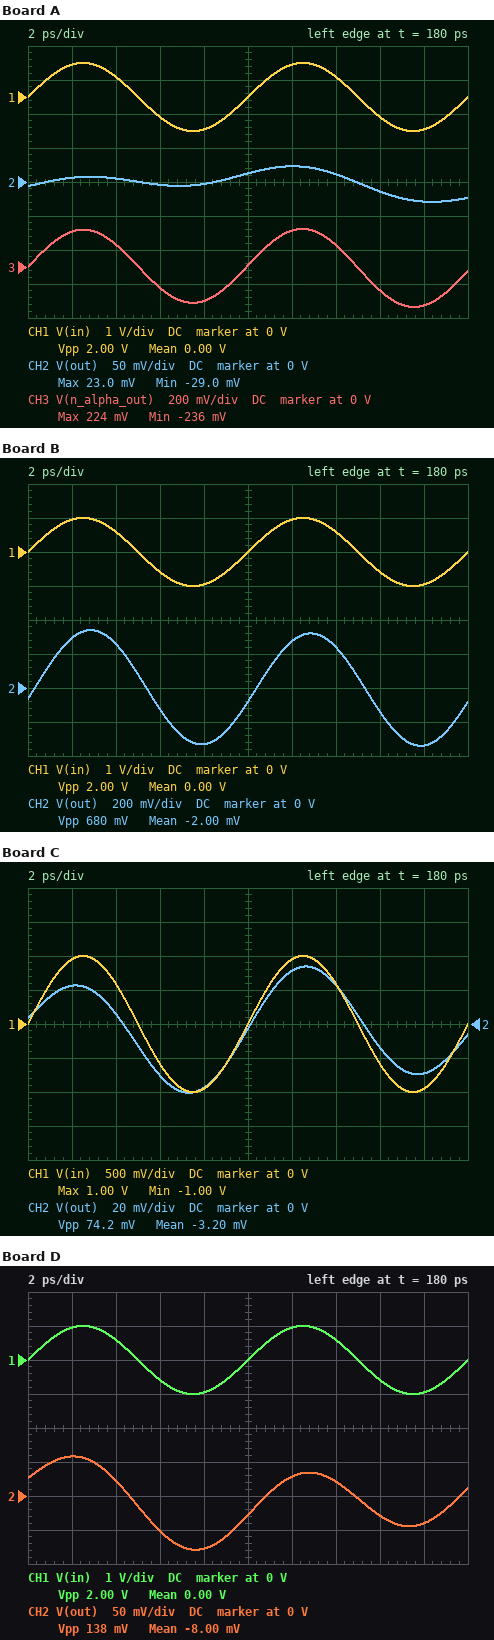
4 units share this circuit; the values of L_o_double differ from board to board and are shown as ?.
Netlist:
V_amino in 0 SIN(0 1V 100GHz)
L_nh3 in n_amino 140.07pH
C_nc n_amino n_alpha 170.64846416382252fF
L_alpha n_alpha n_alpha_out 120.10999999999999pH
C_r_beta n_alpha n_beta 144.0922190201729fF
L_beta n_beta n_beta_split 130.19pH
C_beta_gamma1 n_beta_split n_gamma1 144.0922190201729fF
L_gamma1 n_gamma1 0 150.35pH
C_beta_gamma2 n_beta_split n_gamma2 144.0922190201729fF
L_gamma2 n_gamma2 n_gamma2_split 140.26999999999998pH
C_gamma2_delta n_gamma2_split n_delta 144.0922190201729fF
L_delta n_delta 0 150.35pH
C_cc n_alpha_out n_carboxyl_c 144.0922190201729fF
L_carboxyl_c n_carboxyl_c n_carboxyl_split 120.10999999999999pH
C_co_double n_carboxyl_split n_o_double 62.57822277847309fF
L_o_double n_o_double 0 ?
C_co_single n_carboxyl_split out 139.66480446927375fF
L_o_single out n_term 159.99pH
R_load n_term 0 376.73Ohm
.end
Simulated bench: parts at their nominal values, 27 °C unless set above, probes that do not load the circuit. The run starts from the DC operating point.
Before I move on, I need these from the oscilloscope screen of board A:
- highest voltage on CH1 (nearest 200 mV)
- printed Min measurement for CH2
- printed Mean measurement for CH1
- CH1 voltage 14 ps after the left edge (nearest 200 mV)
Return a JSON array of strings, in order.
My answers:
["1.0 V", "-29.0 mV", "0.00 V", "600 mV"]
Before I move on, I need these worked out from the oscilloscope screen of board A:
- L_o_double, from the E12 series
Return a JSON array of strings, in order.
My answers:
["47 pH"]
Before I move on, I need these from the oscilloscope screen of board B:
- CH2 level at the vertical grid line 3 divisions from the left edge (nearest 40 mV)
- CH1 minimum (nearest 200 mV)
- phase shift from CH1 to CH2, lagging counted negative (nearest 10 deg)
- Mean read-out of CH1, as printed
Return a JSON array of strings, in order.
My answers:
["-120 mV", "-1.0 V", "-10 deg", "0.00 V"]
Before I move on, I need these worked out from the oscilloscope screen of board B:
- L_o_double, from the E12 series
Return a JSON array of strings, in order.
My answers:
["470 pH"]
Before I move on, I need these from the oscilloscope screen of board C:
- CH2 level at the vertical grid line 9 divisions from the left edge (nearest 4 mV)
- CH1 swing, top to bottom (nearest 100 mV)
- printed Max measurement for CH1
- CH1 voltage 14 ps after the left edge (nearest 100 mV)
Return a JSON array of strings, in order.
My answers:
["-28 mV", "2.0 V", "1.00 V", "600 mV"]
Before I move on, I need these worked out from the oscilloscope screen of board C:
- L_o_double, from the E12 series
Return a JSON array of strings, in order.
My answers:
["56 pH"]
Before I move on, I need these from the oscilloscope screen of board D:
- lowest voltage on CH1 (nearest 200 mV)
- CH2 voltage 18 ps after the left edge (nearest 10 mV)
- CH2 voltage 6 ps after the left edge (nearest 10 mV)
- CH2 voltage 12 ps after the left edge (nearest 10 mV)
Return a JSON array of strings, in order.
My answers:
["-1.0 V", "-40 mV", "-50 mV", "30 mV"]
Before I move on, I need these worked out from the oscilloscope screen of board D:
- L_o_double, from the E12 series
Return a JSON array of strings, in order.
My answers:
["68 pH"]
